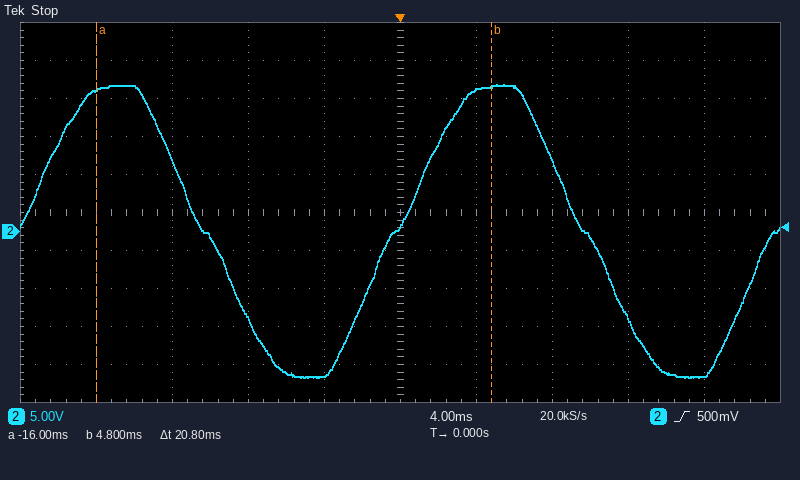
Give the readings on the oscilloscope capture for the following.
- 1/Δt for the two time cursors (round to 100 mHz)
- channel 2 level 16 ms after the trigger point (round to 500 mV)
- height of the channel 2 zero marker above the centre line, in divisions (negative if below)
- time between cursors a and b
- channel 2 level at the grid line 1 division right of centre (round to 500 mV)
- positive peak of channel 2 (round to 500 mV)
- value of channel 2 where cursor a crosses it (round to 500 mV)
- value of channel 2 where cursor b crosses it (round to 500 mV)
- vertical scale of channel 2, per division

48.1 Hz
-19.0 V
-0.5 div
20.8 ms
18.5 V
19.5 V
18.5 V
19.0 V
5 V
